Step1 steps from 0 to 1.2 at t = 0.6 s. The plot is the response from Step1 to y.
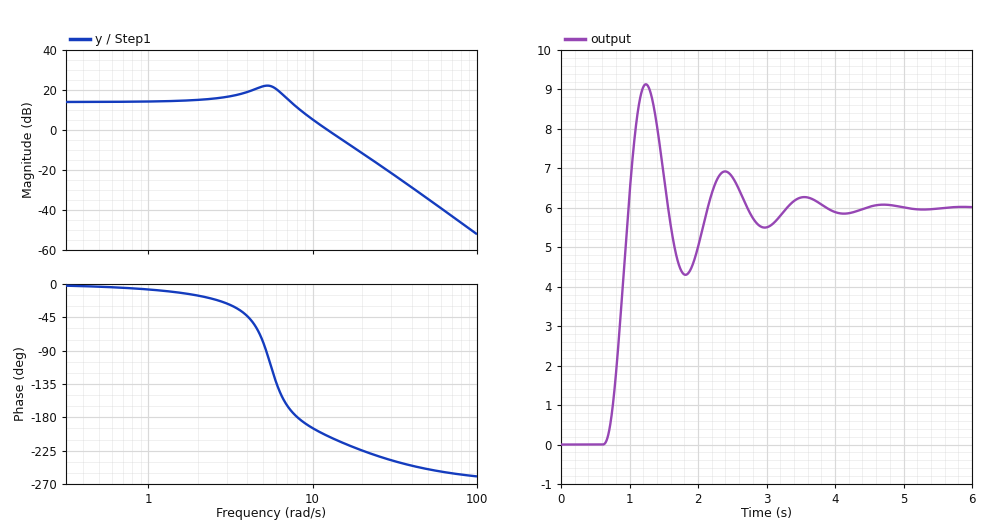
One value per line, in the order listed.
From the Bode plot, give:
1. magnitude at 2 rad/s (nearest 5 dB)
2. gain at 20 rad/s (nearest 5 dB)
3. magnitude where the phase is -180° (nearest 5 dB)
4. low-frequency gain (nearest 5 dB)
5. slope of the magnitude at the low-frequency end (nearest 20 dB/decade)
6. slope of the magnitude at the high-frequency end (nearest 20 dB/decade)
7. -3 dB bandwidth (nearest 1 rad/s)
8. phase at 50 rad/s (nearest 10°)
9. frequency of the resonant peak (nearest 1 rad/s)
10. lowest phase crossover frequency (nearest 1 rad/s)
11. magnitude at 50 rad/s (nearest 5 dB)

15 dB
-10 dB
10 dB
15 dB
0 dB/decade
-60 dB/decade
8 rad/s
-250°
5 rad/s
8 rad/s
-35 dB
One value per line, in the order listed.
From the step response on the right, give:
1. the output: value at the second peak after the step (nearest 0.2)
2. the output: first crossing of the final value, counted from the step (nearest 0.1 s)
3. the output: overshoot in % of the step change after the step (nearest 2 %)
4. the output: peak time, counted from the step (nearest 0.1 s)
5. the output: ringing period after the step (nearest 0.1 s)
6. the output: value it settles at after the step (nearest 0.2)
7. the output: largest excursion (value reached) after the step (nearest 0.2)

7.0
0.4 s
52 %
0.6 s
1.2 s
6.0
9.2
